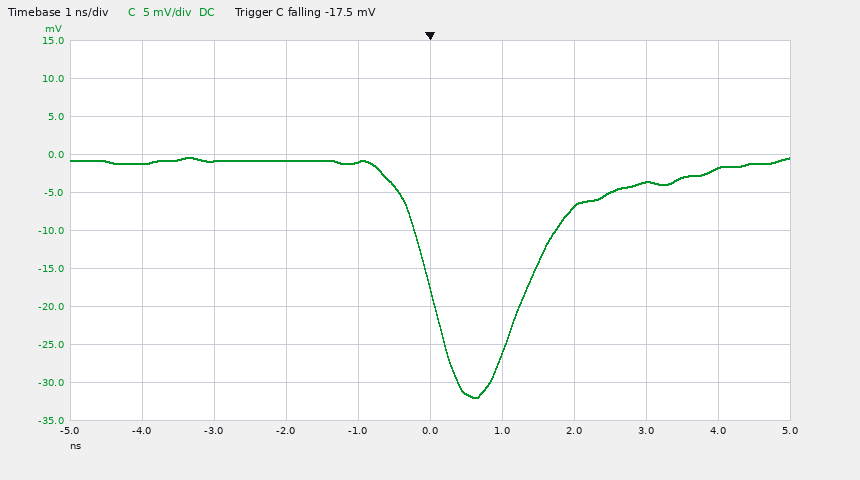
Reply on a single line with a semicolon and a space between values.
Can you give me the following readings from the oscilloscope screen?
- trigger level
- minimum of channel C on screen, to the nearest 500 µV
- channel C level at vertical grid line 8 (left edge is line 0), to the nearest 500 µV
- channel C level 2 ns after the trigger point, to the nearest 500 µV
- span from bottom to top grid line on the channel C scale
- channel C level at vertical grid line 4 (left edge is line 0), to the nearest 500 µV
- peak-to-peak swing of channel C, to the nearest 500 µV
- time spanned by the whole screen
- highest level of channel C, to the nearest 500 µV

-17.5 mV; -32.0 mV; -3.5 mV; -7.0 mV; 50 mV; -1.0 mV; 31.5 mV; 10 ns; -500 µV
